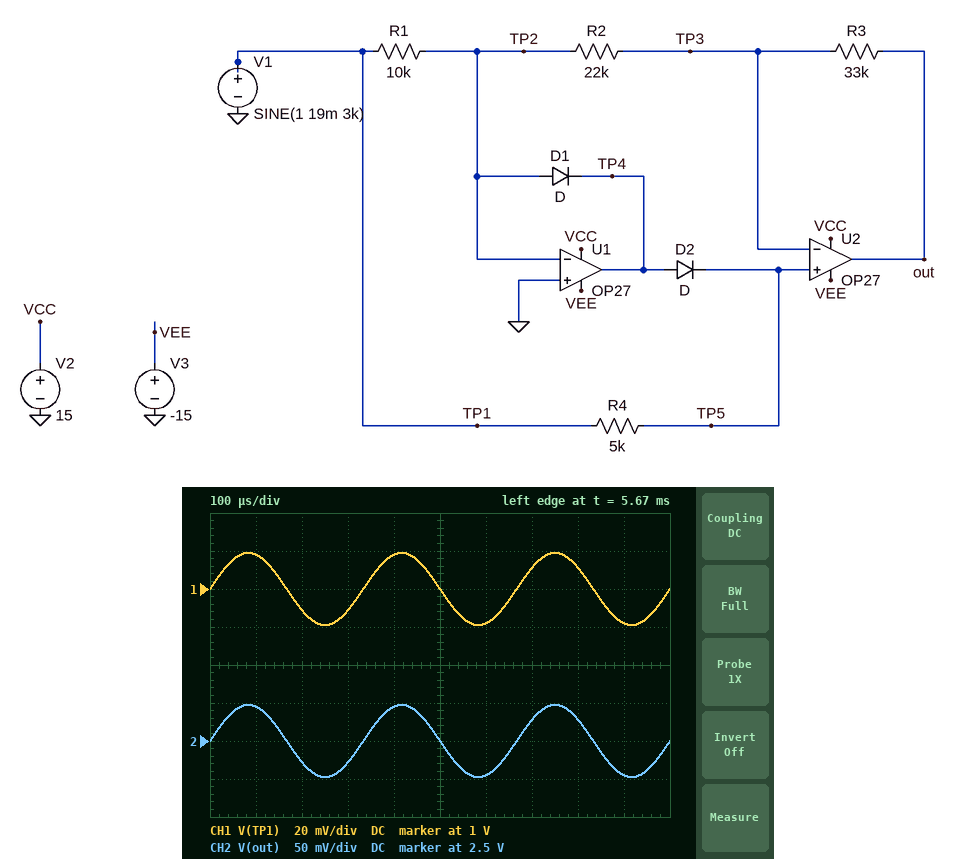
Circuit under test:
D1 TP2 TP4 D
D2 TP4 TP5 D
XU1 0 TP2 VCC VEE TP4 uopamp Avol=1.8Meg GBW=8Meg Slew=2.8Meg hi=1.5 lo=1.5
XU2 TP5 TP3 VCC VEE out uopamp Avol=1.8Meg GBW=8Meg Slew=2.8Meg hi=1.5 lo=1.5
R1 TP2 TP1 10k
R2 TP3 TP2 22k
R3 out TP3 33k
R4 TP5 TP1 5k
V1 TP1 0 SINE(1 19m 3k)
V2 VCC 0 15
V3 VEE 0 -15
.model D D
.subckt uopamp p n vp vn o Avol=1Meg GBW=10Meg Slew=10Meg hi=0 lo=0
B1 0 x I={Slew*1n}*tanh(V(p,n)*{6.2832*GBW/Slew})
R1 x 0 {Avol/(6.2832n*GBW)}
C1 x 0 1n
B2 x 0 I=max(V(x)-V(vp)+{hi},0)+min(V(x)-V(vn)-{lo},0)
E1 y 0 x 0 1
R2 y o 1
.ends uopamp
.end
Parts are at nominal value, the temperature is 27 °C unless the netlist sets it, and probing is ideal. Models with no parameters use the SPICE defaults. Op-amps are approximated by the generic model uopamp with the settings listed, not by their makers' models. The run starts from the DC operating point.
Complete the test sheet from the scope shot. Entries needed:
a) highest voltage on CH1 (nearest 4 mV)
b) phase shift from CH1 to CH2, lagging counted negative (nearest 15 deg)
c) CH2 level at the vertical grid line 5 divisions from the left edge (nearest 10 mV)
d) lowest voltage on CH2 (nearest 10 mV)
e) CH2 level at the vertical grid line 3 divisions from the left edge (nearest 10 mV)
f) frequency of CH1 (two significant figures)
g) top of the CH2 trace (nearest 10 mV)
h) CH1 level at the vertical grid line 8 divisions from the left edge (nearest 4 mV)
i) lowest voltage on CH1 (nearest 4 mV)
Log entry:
1.020 V
0 deg
2.50 V
2.45 V
2.47 V
3.0 kHz
2.55 V
1.012 V
980 mV
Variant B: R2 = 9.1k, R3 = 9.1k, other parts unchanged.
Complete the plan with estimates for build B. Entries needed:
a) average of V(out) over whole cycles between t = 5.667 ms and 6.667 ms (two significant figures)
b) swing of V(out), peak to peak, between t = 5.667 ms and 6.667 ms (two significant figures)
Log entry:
2.0 V
76 mV
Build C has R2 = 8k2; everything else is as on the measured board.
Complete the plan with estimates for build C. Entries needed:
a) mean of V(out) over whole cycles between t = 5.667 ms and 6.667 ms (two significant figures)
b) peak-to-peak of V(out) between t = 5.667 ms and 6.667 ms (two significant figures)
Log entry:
5.0 V
190 mV
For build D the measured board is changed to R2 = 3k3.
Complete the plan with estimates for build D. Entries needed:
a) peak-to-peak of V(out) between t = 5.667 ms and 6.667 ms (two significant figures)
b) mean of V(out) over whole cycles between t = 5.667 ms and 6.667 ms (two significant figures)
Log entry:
420 mV
11 V
